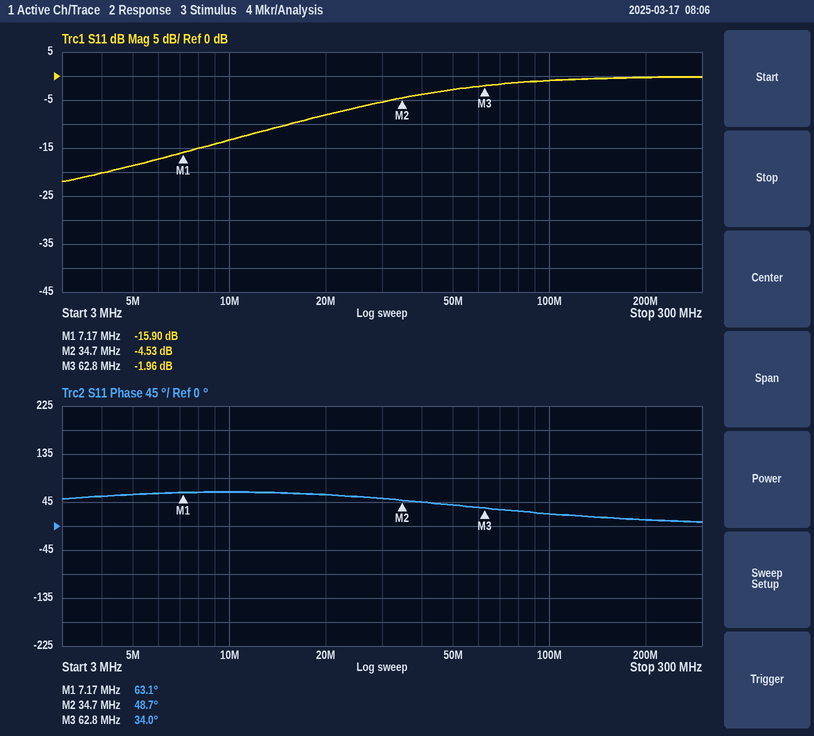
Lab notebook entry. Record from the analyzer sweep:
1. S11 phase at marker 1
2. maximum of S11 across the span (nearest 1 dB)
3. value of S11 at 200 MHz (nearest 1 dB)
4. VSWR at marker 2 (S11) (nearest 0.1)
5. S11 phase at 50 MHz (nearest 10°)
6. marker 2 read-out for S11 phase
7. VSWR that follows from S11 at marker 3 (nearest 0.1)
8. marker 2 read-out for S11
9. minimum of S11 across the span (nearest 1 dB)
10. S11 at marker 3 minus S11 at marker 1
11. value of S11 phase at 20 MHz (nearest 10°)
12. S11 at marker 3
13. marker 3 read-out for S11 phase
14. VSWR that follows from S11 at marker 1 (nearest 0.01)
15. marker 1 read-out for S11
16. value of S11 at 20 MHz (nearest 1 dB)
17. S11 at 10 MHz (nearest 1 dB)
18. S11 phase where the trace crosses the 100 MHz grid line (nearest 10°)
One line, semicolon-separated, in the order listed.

63.1°; 0 dB; 0 dB; 3.9; 40°; 48.7°; 8.9; -4.53 dB; -22 dB; 13.94 dB; 60°; -1.96 dB; 34.0°; 1.38; -15.90 dB; -8 dB; -13 dB; 20°
